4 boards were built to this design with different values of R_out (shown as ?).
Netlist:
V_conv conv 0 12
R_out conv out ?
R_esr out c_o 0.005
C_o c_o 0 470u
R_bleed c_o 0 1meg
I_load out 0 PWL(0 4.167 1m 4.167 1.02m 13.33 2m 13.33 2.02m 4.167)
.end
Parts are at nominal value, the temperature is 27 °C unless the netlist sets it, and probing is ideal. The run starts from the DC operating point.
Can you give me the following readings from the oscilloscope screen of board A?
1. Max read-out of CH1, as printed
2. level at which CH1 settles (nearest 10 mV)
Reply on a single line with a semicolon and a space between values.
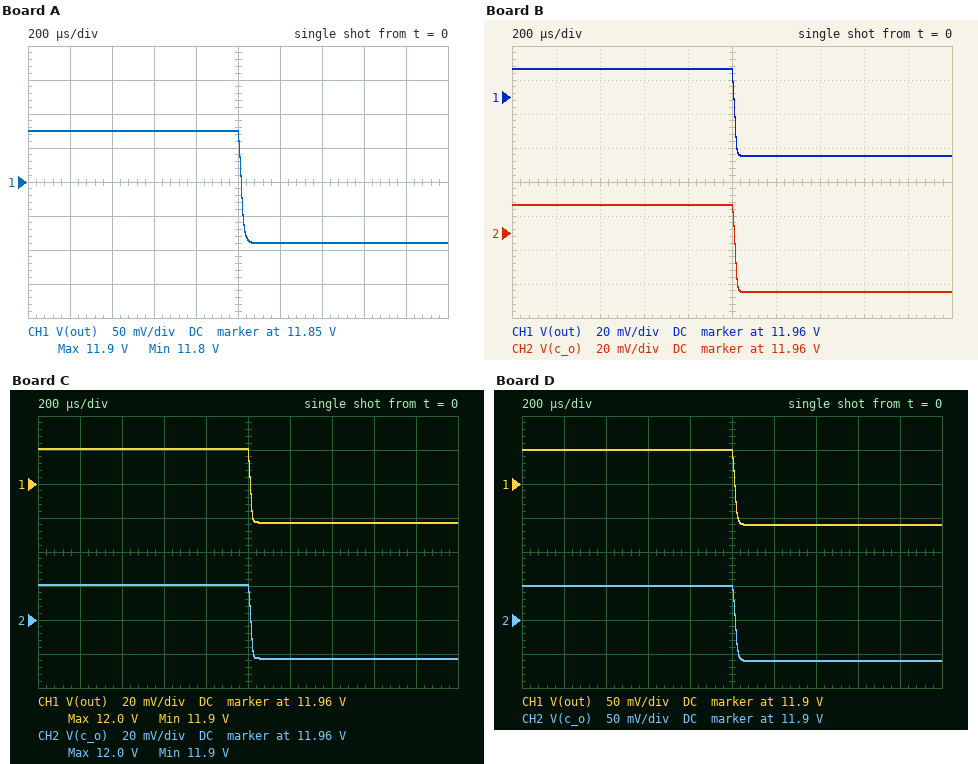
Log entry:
11.9 V; 11.76 V
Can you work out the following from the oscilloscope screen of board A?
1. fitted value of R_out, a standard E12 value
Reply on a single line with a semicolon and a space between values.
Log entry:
0.018 Ω
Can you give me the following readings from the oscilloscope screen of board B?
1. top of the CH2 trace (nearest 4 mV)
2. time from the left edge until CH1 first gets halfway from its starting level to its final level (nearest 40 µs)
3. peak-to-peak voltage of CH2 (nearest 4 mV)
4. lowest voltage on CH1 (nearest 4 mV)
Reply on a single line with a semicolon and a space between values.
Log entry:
11.976 V; 1.00 ms; 52 mV; 11.924 V
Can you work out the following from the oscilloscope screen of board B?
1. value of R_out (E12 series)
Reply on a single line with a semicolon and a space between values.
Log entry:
5.6 mΩ
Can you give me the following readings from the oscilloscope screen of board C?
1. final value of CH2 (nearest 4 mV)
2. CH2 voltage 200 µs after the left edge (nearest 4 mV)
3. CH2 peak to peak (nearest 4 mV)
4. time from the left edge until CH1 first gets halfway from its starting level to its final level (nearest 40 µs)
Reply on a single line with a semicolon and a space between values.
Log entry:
11.936 V; 11.980 V; 44 mV; 1.00 ms
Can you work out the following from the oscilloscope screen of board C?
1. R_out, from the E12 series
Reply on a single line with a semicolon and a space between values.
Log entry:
4.7 mΩ
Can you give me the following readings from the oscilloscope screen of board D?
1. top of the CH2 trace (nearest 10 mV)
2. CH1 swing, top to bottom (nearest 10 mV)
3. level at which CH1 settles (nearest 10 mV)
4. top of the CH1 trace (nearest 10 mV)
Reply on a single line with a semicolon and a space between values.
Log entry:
11.95 V; 110 mV; 11.84 V; 11.95 V
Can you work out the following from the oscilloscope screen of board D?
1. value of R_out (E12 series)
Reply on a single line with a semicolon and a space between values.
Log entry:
0.012 Ω
